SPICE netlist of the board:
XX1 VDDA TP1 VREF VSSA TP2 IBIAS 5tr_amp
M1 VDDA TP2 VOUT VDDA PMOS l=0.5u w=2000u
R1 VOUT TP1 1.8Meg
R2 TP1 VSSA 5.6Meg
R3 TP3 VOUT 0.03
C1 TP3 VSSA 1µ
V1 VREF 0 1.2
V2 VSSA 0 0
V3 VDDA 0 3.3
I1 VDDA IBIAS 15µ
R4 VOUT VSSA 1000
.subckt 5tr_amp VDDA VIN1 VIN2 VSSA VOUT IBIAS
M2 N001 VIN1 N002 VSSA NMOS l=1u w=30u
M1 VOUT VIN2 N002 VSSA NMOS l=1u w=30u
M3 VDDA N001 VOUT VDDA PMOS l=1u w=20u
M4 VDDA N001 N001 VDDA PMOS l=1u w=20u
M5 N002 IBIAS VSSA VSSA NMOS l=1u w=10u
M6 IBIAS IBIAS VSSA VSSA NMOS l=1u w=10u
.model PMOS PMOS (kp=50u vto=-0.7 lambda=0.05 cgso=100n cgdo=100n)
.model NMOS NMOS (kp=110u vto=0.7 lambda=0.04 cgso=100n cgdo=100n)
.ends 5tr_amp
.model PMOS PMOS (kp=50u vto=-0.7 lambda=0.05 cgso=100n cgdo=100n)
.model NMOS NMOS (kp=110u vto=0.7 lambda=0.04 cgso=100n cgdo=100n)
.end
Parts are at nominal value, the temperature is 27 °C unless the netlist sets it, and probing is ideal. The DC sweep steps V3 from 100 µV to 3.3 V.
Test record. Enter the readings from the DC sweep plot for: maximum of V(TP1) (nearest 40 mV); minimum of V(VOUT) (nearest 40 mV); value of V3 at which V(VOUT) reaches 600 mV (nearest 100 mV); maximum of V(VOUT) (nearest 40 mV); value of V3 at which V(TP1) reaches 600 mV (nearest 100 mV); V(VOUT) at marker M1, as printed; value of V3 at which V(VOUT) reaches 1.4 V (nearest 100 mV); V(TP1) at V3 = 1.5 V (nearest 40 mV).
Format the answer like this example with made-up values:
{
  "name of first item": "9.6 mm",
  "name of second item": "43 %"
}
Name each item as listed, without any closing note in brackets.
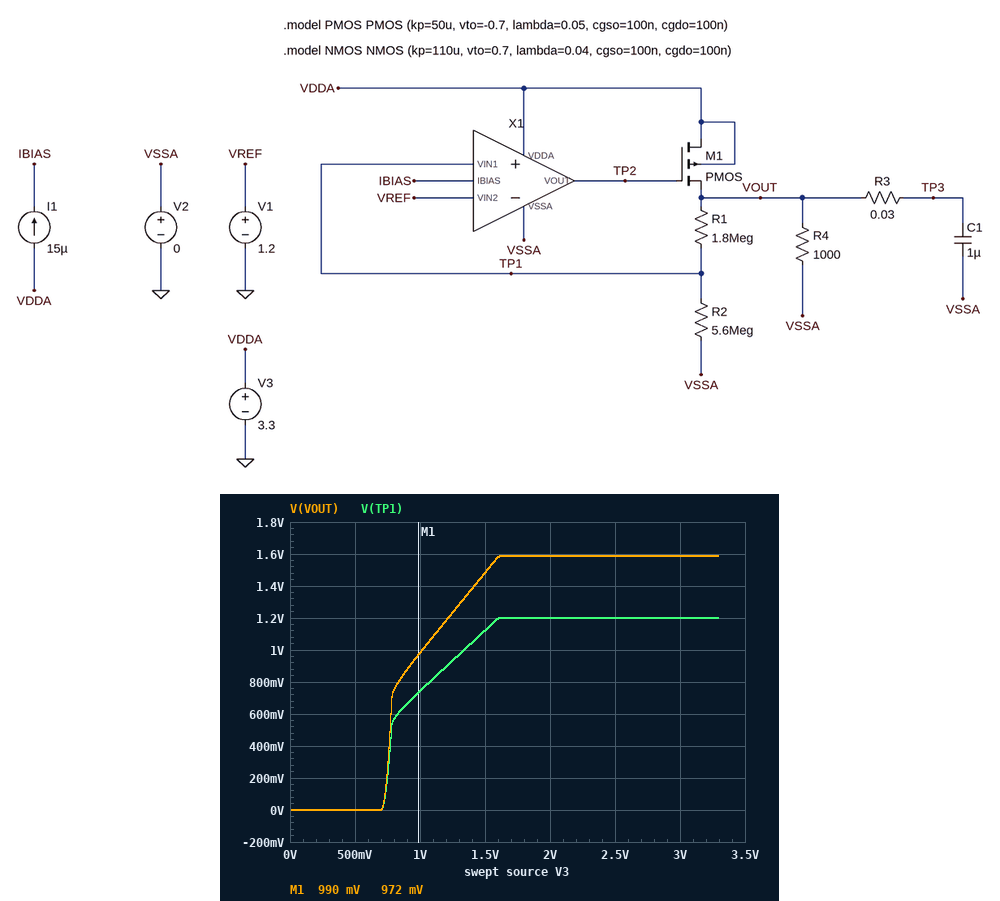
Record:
{
  "maximum of V(TP1)": "1.20 V",
  "minimum of V(VOUT)": "0 V",
  "value of V3 at which V(VOUT) reaches 600 mV": "800 mV",
  "maximum of V(VOUT)": "1.60 V",
  "value of V3 at which V(TP1) reaches 600 mV": "800 mV",
  "V(VOUT) at marker M1, as printed": "972 mV",
  "value of V3 at which V(VOUT) reaches 1.4 V": "1.4 V",
  "V(TP1) at V3 = 1.5 V": "1.12 V"
}
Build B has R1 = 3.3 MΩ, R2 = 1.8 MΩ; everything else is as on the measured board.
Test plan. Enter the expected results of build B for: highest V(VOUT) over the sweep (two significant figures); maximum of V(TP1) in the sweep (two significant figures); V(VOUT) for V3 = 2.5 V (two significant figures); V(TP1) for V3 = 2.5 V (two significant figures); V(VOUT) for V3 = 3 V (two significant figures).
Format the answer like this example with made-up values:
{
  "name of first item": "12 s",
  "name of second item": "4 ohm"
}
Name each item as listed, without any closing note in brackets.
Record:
{
  "highest V(VOUT) over the sweep": "3.3 V",
  "maximum of V(TP1) in the sweep": "1.2 V",
  "V(VOUT) for V3 = 2.5 V": "2.5 V",
  "V(TP1) for V3 = 2.5 V": "880 mV",
  "V(VOUT) for V3 = 3 V": "3.0 V"
}
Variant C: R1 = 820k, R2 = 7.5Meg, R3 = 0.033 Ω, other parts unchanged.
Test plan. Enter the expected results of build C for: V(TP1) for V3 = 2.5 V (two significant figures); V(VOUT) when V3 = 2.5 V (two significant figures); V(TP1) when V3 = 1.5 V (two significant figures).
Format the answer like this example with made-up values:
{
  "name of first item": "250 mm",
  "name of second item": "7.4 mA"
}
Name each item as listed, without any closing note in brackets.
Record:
{
  "V(TP1) for V3 = 2.5 V": "1.2 V",
  "V(VOUT) when V3 = 2.5 V": "1.3 V",
  "V(TP1) when V3 = 1.5 V": "1.2 V"
}
